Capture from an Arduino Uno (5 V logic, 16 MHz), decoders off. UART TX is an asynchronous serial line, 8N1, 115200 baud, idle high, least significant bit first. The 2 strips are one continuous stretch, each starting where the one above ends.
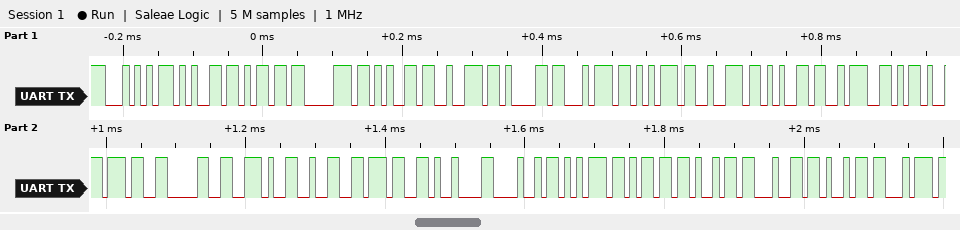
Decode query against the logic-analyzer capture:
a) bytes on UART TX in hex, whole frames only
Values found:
0x54 0x65 0x6D 0x70 0x65 0x72 0x61 0x74 0x75 0x72 0x65 0x3A 0x2D 0x37 0x30 0x2E 0x32 0x37 0x09 0x48 0x75 0x6D 0x69 0x64 0x69 0x74
